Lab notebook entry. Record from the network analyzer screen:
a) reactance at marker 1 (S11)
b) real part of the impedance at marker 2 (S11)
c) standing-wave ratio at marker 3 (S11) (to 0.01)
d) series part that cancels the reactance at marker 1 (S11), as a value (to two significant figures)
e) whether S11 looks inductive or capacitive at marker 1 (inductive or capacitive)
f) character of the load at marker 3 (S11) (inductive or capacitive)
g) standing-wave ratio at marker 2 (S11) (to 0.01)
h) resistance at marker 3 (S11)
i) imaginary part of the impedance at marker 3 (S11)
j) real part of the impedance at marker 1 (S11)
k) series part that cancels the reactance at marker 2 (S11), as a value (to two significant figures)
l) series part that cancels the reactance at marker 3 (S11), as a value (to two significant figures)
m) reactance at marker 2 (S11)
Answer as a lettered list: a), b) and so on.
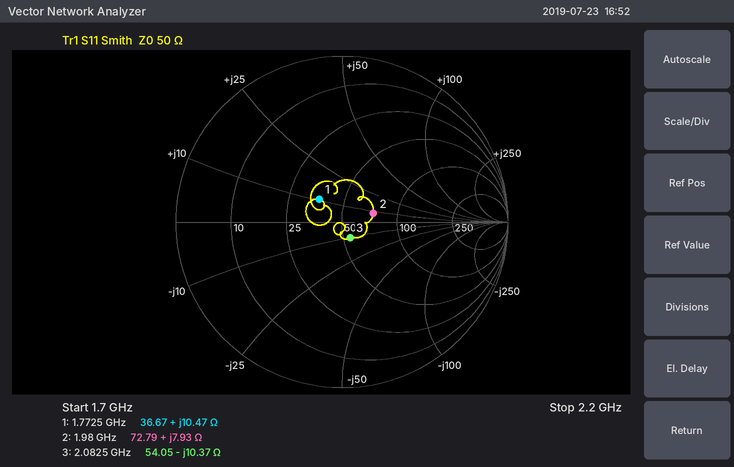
a) +10.47 Ω
b) 72.79 Ω
c) 1.24
d) 8.6 pF
e) inductive
f) capacitive
g) 1.49
h) 54.05 Ω
i) -10.37 Ω
j) 36.67 Ω
k) 10 pF
l) 790 pH
m) +7.93 Ω
